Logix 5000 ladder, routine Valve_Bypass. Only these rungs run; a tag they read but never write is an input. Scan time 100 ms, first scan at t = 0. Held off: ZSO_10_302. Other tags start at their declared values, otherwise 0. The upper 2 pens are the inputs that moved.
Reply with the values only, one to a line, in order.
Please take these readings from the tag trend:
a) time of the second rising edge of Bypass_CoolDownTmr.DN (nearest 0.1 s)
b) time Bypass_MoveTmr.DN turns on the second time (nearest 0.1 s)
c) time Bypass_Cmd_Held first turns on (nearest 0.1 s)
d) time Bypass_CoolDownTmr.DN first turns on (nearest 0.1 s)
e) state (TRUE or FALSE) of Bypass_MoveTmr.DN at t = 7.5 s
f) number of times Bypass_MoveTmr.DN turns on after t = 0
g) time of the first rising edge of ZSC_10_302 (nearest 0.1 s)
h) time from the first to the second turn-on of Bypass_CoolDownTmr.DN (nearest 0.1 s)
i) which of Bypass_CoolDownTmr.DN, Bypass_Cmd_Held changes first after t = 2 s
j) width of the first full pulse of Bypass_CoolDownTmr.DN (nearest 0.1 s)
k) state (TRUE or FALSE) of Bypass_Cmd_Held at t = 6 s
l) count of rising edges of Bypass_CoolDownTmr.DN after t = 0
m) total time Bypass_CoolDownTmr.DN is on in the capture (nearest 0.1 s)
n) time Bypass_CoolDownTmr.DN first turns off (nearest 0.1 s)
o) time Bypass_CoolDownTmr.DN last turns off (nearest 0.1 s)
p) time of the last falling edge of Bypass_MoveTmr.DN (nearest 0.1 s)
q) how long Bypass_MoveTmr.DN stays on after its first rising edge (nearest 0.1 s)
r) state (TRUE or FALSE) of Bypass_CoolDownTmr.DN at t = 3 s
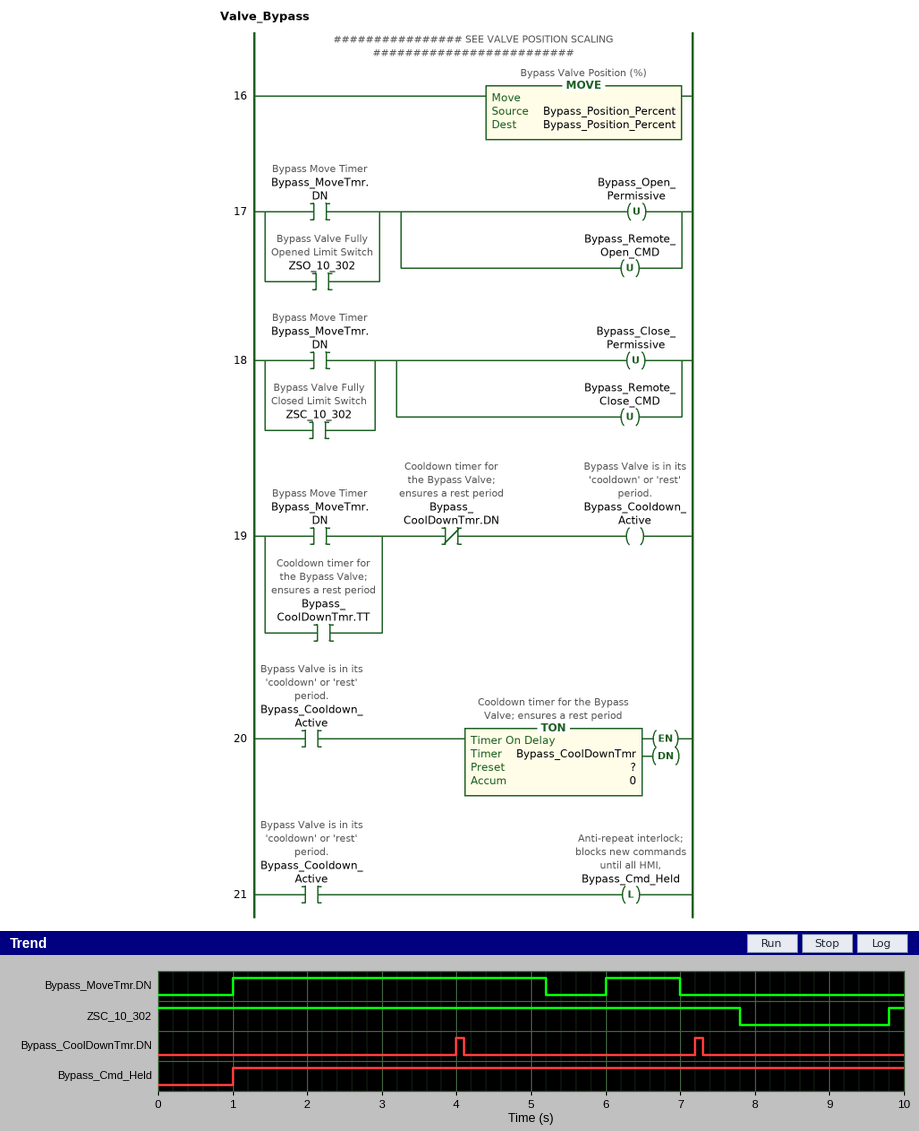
7.2 s
6.0 s
1.0 s
4.0 s
FALSE
2
9.8 s
3.2 s
Bypass_CoolDownTmr.DN
0.1 s
TRUE
2
0.2 s
4.1 s
7.3 s
7.0 s
4.2 s
FALSE
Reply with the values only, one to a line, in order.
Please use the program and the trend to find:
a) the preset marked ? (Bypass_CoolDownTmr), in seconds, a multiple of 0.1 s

3.0 s
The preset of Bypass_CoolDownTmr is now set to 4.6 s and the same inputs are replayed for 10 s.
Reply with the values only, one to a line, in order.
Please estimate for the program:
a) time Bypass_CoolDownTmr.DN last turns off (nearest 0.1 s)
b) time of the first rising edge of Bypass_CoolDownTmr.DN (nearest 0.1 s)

5.7 s
5.6 s
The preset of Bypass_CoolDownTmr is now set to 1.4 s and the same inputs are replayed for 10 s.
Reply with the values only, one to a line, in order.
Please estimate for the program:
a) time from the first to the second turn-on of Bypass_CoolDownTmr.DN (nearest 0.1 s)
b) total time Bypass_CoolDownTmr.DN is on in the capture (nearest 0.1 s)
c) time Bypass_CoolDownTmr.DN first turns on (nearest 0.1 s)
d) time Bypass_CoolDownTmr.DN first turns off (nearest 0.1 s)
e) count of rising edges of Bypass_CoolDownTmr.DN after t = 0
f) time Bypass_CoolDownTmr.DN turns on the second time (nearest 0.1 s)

1.6 s
0.4 s
2.4 s
2.5 s
4
4.0 s
